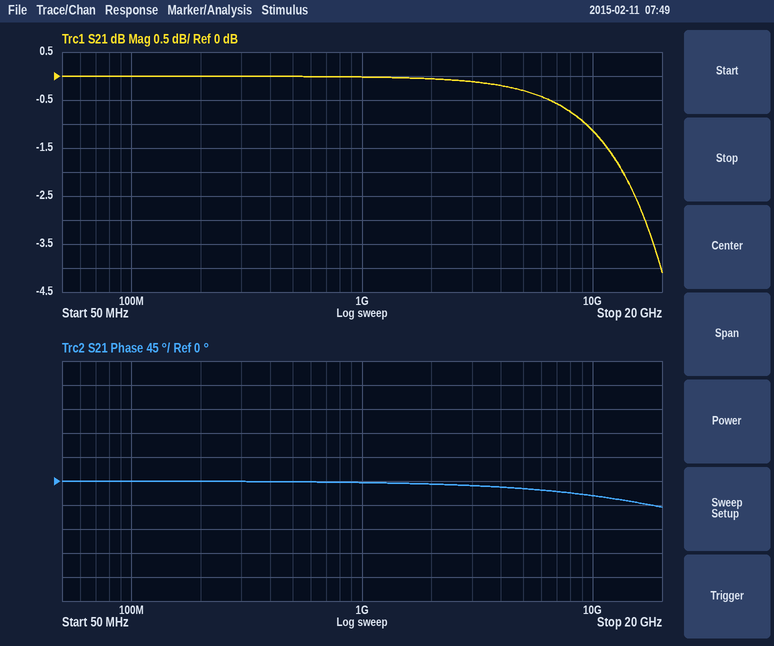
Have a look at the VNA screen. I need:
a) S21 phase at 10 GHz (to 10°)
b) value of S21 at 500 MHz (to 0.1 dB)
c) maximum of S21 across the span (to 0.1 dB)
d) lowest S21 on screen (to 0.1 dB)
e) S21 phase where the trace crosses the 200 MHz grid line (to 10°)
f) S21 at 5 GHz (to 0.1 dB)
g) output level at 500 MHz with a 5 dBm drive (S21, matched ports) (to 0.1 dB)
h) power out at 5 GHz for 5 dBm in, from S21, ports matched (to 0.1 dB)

-30°
0.0 dB
0.0 dB
-4.1 dB
0°
-0.3 dB
5.0 dBm
4.7 dBm
